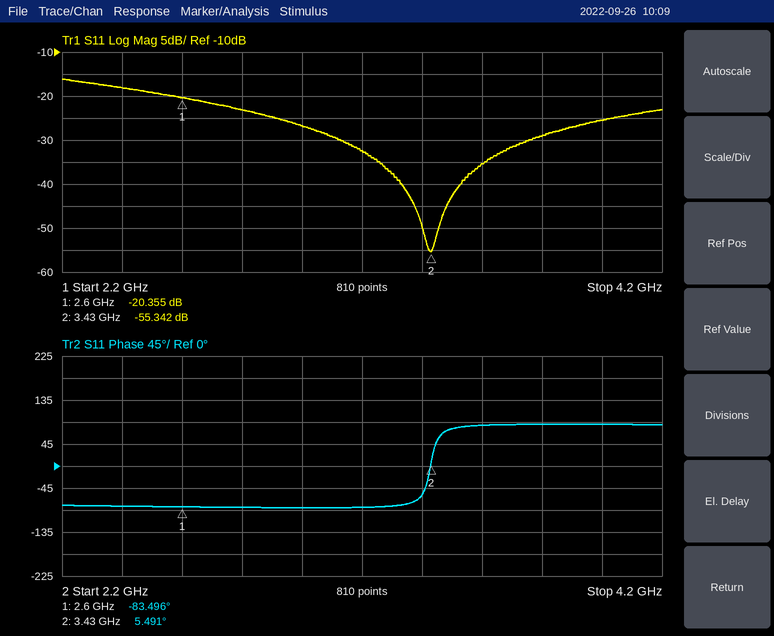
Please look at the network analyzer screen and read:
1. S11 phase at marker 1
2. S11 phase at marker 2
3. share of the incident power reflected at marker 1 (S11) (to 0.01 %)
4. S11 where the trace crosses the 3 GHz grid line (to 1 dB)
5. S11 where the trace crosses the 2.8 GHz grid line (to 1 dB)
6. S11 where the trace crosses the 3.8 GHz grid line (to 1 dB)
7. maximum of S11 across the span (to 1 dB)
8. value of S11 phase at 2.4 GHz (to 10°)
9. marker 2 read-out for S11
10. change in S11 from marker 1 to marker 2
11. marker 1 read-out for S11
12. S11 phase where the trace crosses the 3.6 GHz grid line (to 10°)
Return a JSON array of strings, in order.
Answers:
["-83.496°", "5.491°", "0.92 %", "-27 dB", "-23 dB", "-29 dB", "-16 dB", "-80°", "-55.342 dB", "-34.987 dB", "-20.355 dB", "80°"]
